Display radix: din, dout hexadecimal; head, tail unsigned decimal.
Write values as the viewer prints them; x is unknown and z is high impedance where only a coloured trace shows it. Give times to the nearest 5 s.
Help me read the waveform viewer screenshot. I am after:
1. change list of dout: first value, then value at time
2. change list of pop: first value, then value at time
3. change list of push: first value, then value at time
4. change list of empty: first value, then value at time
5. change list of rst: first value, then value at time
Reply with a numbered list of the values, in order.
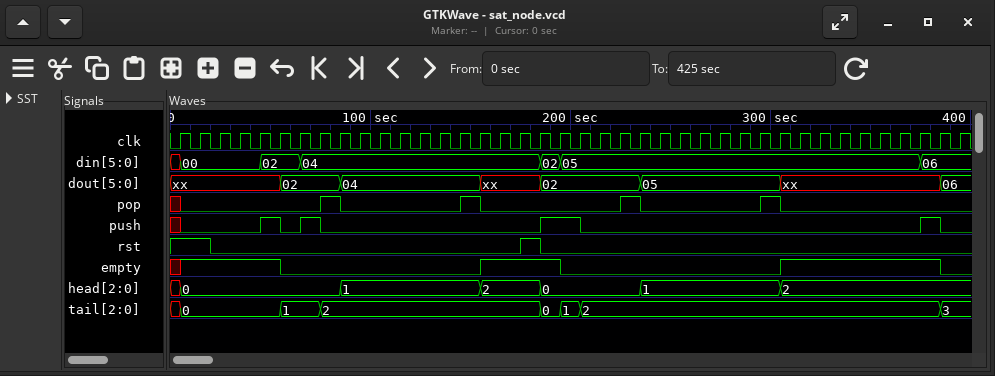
1. xx, 02 at 55 s, 04 at 85 s, xx at 155 s, 02 at 185 s, 05 at 235 s, xx at 305 s, 06 at 385 s
2. x, 0 at 5 s, 1 at 75 s, 0 at 85 s, 1 at 145 s, 0 at 155 s, 1 at 225 s, 0 at 235 s, 1 at 295 s, 0 at 305 s
3. x, 0 at 5 s, 1 at 45 s, 0 at 55 s, 1 at 65 s, 0 at 75 s, 1 at 185 s, 0 at 205 s, 1 at 375 s, 0 at 385 s
4. x, 1 at 5 s, 0 at 55 s, 1 at 155 s, 0 at 195 s, 1 at 305 s, 0 at 385 s
5. 1, 0 at 20 s, 1 at 175 s, 0 at 185 s
